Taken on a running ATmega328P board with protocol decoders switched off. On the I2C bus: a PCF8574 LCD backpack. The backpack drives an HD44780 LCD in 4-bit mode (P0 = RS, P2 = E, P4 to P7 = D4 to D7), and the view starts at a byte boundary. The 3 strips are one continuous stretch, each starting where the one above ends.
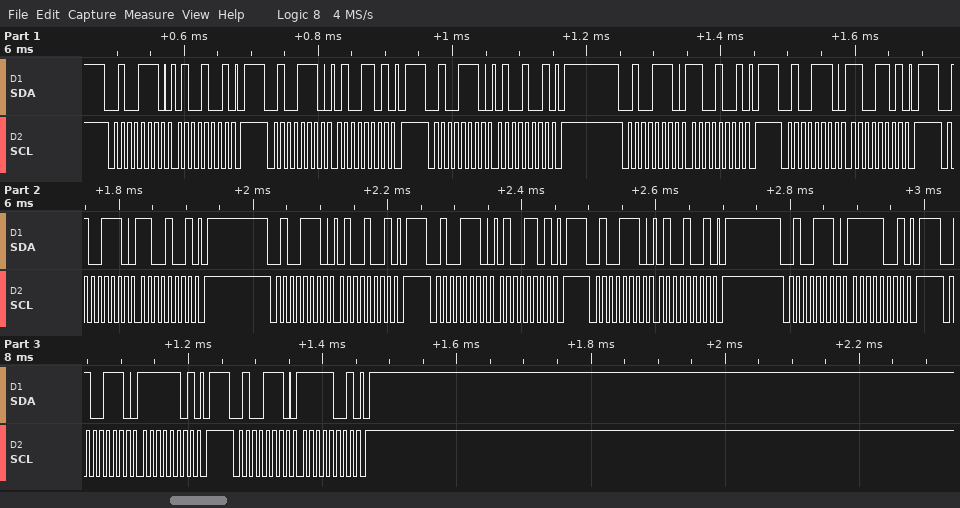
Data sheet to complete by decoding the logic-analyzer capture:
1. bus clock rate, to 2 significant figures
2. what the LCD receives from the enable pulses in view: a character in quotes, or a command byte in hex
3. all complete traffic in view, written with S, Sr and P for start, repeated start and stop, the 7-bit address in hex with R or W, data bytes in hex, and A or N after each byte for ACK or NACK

100 kHz
'L' 'O'
S 27W A 49 A P S 27W A 4D A P S 27W A 49 A P S 27W A C9 A P S 27W A CD A P S 27W A C9 A P S 27W A 49 A P S 27W A 4D A P S 27W A 49 A P S 27W A F9 A P S 27W A FD A P S 27W A F9 A P
